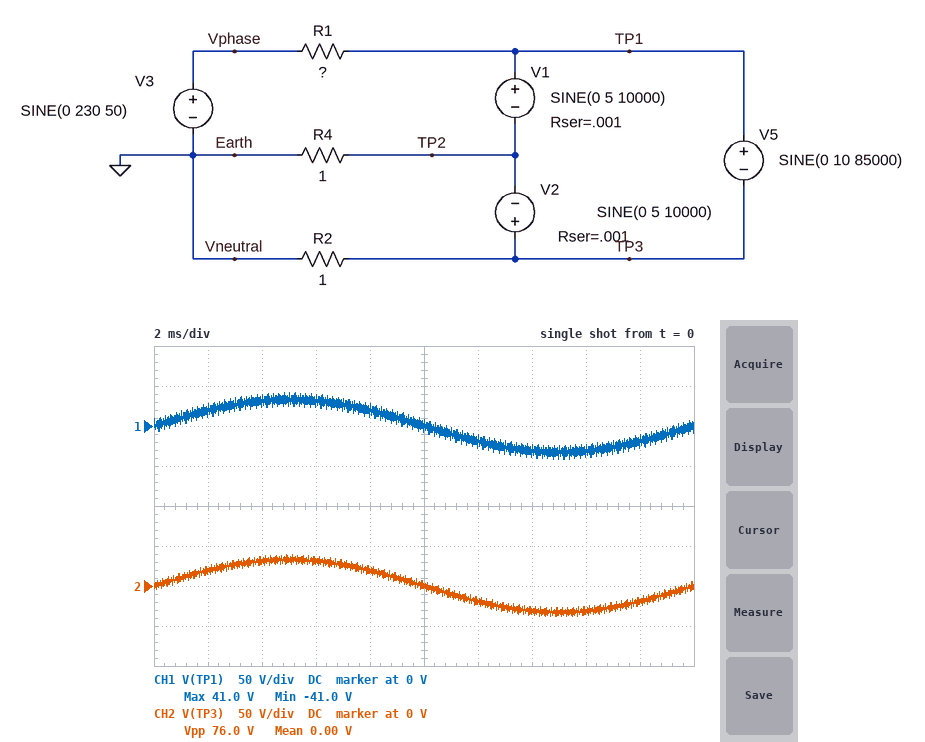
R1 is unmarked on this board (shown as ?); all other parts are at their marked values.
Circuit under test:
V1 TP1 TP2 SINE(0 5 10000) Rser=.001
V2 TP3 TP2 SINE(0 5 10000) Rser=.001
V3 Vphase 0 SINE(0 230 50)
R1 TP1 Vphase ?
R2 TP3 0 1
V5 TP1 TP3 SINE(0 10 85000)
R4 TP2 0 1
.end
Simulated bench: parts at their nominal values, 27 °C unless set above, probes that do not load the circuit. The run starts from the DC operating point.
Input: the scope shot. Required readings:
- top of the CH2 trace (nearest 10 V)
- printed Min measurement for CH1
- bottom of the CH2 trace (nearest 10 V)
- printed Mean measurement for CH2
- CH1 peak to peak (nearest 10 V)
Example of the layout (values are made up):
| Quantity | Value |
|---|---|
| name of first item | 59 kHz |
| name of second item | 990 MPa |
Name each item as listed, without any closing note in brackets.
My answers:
| Quantity | Value |
|---|---|
| top of the CH2 trace | 40 V |
| printed Min measurement for CH1 | -41.0 V |
| bottom of the CH2 trace | -40 V |
| printed Mean measurement for CH2 | 0.00 V |
| CH1 peak to peak | 80 V |
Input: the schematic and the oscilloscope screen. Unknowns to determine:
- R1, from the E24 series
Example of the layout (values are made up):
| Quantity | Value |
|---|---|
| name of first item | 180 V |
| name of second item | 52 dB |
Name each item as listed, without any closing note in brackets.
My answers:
| Quantity | Value |
|---|---|
| R1, from the E24 series | 3 Ω |
